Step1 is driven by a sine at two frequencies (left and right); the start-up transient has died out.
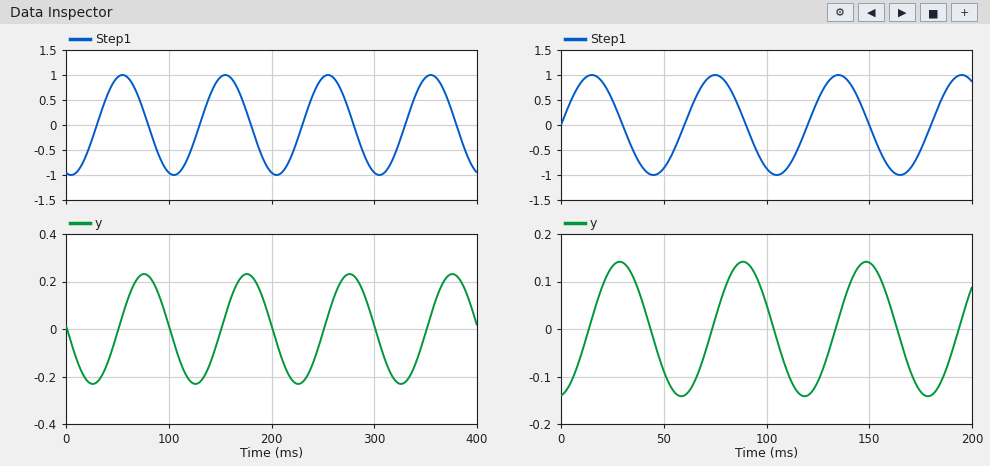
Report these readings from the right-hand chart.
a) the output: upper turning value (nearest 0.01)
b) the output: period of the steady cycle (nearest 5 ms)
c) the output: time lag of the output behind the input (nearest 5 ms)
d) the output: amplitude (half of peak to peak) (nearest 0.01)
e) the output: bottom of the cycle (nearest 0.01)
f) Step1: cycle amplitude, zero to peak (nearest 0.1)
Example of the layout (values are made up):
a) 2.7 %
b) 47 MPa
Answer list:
a) 0.14
b) 60 ms
c) 15 ms
d) 0.14
e) -0.14
f) 1.0
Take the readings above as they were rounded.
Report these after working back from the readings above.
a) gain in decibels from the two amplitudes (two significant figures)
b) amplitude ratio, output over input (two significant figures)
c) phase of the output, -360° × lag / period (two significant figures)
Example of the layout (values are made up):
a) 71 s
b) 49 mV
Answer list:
a) -17 dB
b) 0.14
c) -90°
